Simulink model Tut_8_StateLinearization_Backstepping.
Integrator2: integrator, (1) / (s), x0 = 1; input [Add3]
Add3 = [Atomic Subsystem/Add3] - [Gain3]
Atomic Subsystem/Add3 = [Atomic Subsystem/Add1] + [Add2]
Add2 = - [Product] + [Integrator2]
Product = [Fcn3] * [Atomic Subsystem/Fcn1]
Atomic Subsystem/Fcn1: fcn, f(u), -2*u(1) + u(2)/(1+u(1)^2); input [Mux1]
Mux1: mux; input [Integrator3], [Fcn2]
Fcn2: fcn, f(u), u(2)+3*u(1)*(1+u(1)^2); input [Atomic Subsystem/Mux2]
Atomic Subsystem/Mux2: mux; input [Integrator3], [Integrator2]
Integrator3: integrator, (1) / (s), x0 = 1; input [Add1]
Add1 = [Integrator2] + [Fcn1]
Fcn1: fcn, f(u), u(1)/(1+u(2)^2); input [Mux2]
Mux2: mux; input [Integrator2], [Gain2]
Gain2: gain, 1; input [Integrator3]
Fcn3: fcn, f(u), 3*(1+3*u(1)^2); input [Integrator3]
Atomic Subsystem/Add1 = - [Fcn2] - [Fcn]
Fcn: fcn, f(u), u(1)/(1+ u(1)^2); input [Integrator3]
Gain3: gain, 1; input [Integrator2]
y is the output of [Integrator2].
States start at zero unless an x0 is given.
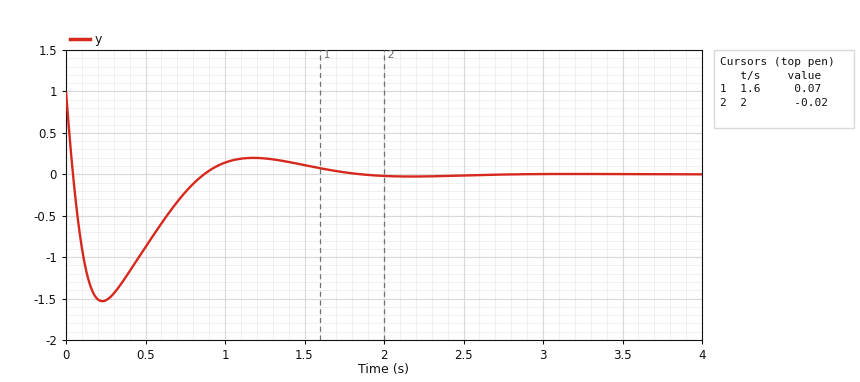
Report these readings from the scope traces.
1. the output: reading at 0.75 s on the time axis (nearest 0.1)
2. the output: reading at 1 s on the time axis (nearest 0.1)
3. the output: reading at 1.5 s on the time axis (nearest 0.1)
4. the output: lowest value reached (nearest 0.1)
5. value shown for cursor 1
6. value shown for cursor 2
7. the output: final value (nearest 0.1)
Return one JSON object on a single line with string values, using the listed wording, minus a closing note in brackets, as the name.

{"the output: reading at 0.75 s on the time axis": "-0.2", "the output: reading at 1 s on the time axis": "0.1", "the output: reading at 1.5 s on the time axis": "0.1", "the output: lowest value reached": "-1.5", "value shown for cursor 1": "0.07", "value shown for cursor 2": "-0.02", "the output: final value": "0.0"}
